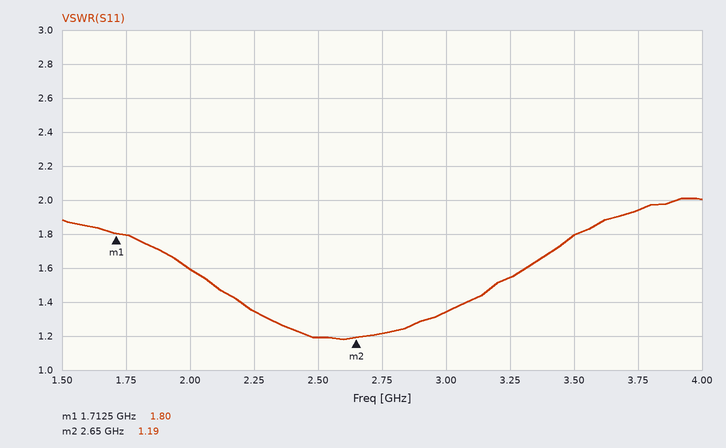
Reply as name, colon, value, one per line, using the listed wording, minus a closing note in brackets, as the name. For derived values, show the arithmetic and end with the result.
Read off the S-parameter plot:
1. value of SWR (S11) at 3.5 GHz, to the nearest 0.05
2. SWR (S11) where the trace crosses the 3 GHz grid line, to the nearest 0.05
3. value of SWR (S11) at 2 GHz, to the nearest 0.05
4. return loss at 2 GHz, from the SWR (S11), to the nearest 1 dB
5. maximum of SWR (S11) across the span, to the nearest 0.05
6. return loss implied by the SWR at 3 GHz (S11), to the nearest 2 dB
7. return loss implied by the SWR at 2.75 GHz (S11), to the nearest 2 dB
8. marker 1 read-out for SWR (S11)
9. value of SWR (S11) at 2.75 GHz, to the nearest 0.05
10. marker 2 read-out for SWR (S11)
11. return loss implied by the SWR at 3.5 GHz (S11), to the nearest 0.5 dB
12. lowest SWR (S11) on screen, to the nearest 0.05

value of SWR (S11) at 3.5 GHz, to the nearest 0.05: 1.80
SWR (S11) where the trace crosses the 3 GHz grid line, to the nearest 0.05: 1.35
value of SWR (S11) at 2 GHz, to the nearest 0.05: 1.60
return loss at 2 GHz, from the SWR (S11), to the nearest 1 dB: −20 log10((1.6 − 1)/(1.6 + 1)) ≈ 13 dB
maximum of SWR (S11) across the span, to the nearest 0.05: 2.00
return loss implied by the SWR at 3 GHz (S11), to the nearest 2 dB: −20 log10((1.35 − 1)/(1.35 + 1)) ≈ 16 dB
return loss implied by the SWR at 2.75 GHz (S11), to the nearest 2 dB: −20 log10((1.2 − 1)/(1.2 + 1)) ≈ 20.8 dB, so 20 dB to the nearest 2 dB
marker 1 read-out for SWR: 1.80
value of SWR (S11) at 2.75 GHz, to the nearest 0.05: 1.20
marker 2 read-out for SWR: 1.19
return loss implied by the SWR at 3.5 GHz (S11), to the nearest 0.5 dB: −20 log10((1.8 − 1)/(1.8 + 1)) ≈ 10.9 dB, so 11.0 dB to the nearest 0.5 dB
lowest SWR (S11) on screen, to the nearest 0.05: 1.20
